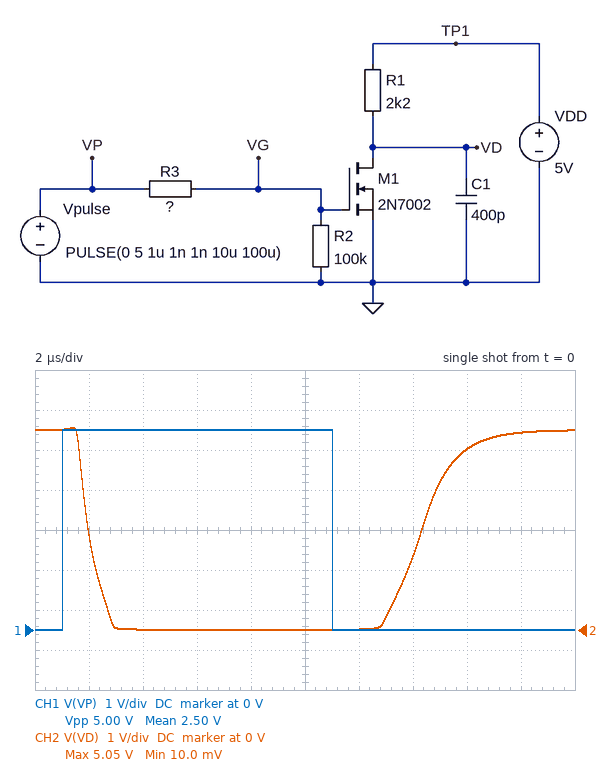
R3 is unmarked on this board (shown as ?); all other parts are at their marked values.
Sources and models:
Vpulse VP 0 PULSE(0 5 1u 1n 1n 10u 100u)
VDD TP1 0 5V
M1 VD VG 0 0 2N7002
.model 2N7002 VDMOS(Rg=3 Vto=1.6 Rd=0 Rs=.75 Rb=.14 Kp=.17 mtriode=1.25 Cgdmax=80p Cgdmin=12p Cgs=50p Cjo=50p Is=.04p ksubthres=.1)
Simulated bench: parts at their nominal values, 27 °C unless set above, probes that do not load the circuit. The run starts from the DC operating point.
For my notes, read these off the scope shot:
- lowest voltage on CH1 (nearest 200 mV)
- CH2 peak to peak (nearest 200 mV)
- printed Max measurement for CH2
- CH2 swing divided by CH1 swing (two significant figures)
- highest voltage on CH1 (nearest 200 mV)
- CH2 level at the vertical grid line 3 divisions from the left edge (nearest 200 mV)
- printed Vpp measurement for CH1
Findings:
0 V
5.0 V
5.05 V
1.0
5.0 V
0 V
5.00 V
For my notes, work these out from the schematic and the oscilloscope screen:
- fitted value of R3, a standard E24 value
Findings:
18 kΩ
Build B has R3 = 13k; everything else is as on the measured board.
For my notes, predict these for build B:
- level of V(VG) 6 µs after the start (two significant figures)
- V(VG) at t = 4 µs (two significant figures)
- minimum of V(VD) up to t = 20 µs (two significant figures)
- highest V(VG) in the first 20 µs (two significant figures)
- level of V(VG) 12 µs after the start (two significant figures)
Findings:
4.2 V
3.5 V
4.8 mV
4.4 V
2.3 V
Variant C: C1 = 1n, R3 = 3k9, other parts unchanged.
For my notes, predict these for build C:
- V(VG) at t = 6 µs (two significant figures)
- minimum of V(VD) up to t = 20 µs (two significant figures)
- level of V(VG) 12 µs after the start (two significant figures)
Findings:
4.8 V
3.0 mV
850 mV
